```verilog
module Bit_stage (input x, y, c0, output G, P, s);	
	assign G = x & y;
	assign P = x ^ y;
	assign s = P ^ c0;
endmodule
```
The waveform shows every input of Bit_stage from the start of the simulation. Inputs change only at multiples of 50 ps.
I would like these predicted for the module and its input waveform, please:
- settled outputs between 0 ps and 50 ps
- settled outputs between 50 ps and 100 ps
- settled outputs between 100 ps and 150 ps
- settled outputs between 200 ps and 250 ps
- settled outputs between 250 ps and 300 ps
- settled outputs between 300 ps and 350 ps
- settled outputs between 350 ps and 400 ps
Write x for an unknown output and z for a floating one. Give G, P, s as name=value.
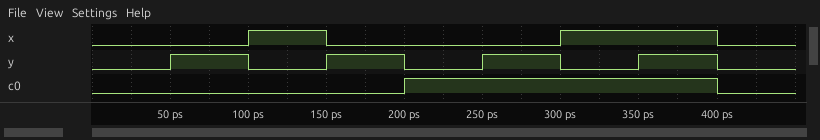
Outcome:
G=0, P=0, s=0
G=0, P=1, s=1
G=0, P=1, s=1
G=0, P=0, s=1
G=0, P=1, s=0
G=0, P=1, s=0
G=1, P=0, s=1
